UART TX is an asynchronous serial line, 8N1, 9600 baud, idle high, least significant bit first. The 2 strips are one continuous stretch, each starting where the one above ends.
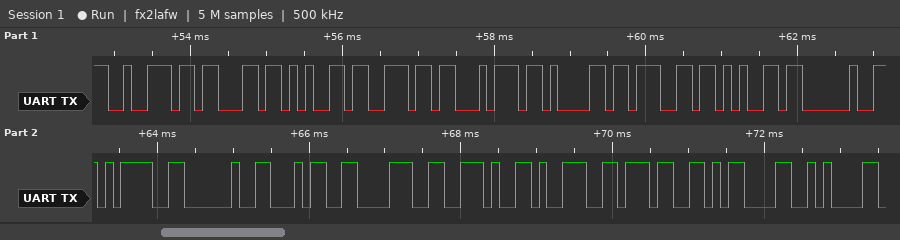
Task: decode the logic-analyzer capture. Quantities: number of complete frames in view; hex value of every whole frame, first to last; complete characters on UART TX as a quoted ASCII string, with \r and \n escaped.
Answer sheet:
18
72 63 65 6E 74 61 67 65 20 3D 20 34 38 2E 39 37 0D 0A
"rcentage = 48.97\r\n"
